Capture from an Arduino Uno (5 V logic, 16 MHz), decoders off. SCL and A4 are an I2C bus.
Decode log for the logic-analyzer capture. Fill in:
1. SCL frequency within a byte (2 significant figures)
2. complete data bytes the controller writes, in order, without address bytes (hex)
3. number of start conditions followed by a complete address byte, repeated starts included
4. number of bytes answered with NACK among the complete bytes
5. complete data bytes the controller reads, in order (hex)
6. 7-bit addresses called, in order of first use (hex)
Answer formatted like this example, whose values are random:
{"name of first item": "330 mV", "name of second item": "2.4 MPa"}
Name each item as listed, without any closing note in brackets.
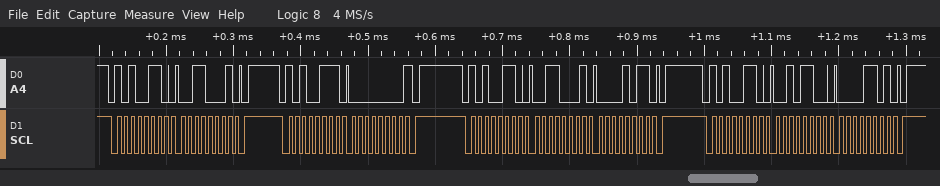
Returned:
{"SCL frequency within a byte": "100 kHz", "complete data bytes the controller writes, in order, without address bytes": "31 31 0B 2C 0D", "number of start conditions followed by a complete address byte, repeated starts included": "4", "number of bytes answered with NACK among the complete bytes": "1", "complete data bytes the controller reads, in order": "00", "7-bit addresses called, in order of first use": "0x53"}
